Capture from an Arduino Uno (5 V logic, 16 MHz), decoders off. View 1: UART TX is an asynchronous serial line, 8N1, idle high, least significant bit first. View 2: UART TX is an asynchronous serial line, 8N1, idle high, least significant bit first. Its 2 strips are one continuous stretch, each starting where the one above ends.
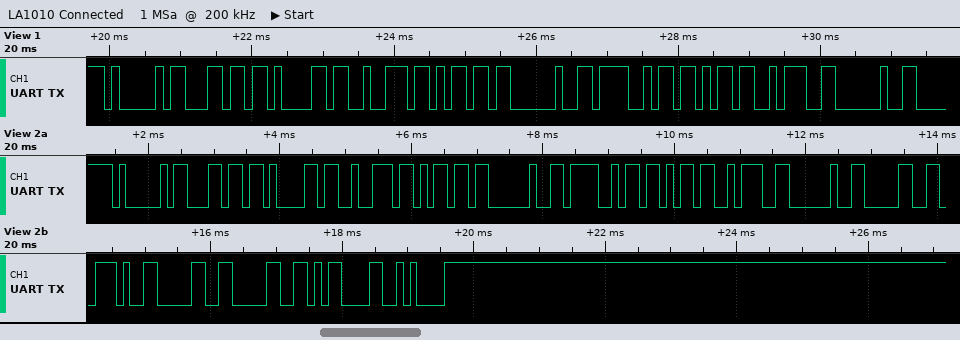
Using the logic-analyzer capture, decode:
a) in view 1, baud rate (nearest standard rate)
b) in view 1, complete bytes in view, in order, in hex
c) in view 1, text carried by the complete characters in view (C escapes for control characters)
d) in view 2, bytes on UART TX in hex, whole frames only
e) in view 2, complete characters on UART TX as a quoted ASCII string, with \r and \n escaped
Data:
9600 baud
0x41 0x6C 0x61 0x72 0x6D 0x20 0x4F 0x6B 0x3A 0x20
"Alarm Ok: "
41 6C 61 72 6D 20 4F 6B 3A 20 30 2E 30 30 0D 0A
"Alarm Ok: 0.00\r\n"
